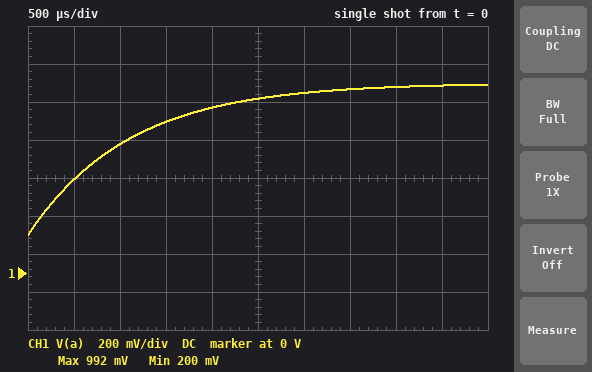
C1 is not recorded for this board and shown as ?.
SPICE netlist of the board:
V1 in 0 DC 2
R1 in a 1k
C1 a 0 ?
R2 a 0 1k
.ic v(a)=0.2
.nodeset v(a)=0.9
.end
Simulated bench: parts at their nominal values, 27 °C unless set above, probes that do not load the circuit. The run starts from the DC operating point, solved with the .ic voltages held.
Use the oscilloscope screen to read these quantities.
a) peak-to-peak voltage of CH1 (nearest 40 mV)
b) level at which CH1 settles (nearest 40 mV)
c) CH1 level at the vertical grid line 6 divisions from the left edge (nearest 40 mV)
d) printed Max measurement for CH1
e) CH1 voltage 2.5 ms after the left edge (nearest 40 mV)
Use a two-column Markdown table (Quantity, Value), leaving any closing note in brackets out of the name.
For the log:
| Quantity | Value |
|---|---|
| peak-to-peak voltage of CH1 | 800 mV |
| level at which CH1 settles | 1.00 V |
| CH1 level at the vertical grid line 6 divisions from the left edge | 960 mV |
| printed Max measurement for CH1 | 992 mV |
| CH1 voltage 2.5 ms after the left edge | 920 mV |
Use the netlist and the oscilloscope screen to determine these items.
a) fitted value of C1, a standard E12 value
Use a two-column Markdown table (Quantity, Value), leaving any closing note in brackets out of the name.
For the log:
| Quantity | Value |
|---|---|
| fitted value of C1, a standard E12 value | 2.2 µF |
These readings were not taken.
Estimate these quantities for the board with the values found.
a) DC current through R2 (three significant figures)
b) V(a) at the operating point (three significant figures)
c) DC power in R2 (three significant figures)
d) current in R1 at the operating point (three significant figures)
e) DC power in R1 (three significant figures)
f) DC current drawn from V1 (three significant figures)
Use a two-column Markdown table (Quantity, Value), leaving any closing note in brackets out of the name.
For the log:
| Quantity | Value |
|---|---|
| DC current through R2 | 1.00 mA |
| V(a) at the operating point | 1.00 V |
| DC power in R2 | 1.00 mW |
| current in R1 at the operating point | 1.00 mA |
| DC power in R1 | 1.00 mW |
| DC current drawn from V1 | 1.00 mA |
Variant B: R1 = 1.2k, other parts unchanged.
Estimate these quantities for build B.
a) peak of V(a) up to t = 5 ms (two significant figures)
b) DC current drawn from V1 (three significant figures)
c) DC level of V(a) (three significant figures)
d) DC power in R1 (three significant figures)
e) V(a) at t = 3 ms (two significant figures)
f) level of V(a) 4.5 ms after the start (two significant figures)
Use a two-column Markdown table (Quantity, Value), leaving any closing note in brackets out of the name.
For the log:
| Quantity | Value |
|---|---|
| peak of V(a) up to t = 5 ms | 900 mV |
| DC current drawn from V1 | 909 µA |
| DC level of V(a) | 909 mV |
| DC power in R1 | 992 µW |
| V(a) at t = 3 ms | 850 mV |
| level of V(a) 4.5 ms after the start | 890 mV |
